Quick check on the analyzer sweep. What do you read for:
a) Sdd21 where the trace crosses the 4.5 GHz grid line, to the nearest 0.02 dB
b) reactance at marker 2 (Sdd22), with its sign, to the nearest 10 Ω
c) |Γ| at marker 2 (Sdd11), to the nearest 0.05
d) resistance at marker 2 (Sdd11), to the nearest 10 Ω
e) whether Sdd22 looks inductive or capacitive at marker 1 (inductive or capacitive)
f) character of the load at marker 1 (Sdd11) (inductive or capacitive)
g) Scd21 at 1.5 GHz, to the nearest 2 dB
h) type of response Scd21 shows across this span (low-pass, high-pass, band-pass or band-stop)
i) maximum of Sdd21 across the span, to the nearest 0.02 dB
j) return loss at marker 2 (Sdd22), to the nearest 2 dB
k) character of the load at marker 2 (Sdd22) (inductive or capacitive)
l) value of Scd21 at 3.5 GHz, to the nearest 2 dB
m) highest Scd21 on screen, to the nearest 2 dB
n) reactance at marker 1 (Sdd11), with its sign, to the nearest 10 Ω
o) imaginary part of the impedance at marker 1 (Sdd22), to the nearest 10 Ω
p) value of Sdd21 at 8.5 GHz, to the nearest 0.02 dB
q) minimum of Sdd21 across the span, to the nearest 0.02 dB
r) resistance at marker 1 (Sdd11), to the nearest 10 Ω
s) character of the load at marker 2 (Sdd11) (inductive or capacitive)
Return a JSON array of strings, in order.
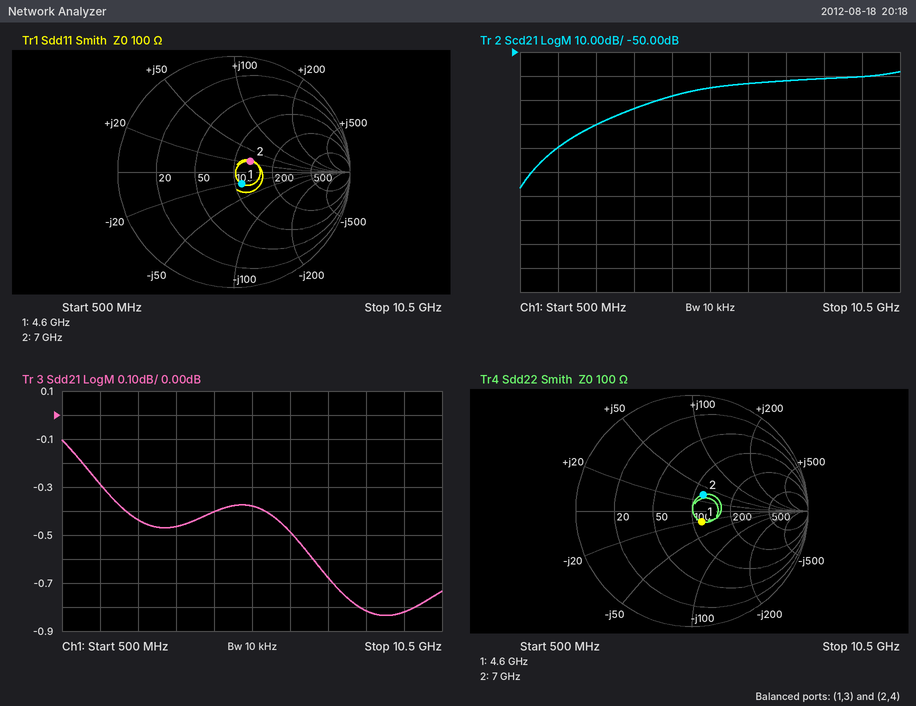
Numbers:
["-0.40 dB", "+30 Ω", "0.15", "130 Ω", "capacitive", "capacitive", "-90 dB", "high-pass", "-0.10 dB", "16 dB", "inductive", "-74 dB", "-58 dB", "-20 Ω", "-20 Ω", "-0.82 dB", "-0.84 dB", "110 Ω", "inductive"]
